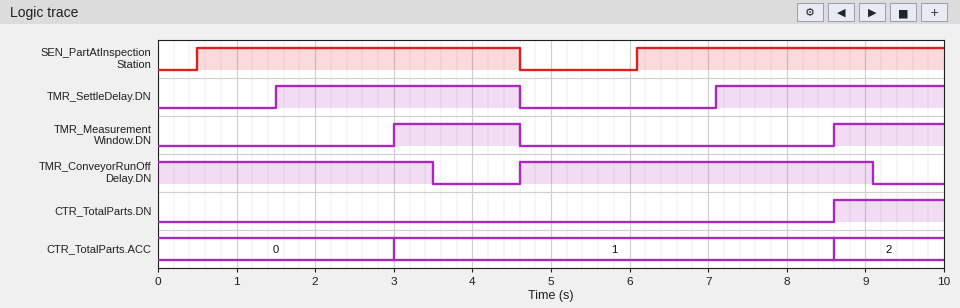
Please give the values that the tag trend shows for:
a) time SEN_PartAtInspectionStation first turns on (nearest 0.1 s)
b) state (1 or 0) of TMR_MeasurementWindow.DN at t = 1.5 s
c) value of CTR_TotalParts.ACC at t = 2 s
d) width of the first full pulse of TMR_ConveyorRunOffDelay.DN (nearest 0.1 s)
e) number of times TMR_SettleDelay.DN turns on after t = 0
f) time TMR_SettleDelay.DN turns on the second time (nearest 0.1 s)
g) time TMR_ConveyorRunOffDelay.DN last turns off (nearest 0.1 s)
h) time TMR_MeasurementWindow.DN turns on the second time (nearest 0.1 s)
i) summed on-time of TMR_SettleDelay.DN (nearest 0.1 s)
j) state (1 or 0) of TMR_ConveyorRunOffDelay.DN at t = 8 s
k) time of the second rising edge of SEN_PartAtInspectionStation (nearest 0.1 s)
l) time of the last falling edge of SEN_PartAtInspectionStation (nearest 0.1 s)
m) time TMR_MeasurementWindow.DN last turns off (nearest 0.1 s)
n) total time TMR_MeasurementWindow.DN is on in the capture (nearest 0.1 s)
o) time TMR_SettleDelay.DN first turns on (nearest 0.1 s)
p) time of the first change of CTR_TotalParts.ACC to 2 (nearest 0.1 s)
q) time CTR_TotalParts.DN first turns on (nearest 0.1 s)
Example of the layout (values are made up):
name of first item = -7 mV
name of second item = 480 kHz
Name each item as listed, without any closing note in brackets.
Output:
time SEN_PartAtInspectionStation first turns on = 0.5 s
state (1 or 0) of TMR_MeasurementWindow.DN at t = 1.5 s = 0
value of CTR_TotalParts.ACC at t = 2 s = 0
width of the first full pulse of TMR_ConveyorRunOffDelay.DN = 4.5 s
number of times TMR_SettleDelay.DN turns on after t = 0 = 2
time TMR_SettleDelay.DN turns on the second time = 7.1 s
time TMR_ConveyorRunOffDelay.DN last turns off = 9.1 s
time TMR_MeasurementWindow.DN turns on the second time = 8.6 s
summed on-time of TMR_SettleDelay.DN = 6.0 s
state (1 or 0) of TMR_ConveyorRunOffDelay.DN at t = 8 s = 1
time of the second rising edge of SEN_PartAtInspectionStation = 6.1 s
time of the last falling edge of SEN_PartAtInspectionStation = 4.6 s
time TMR_MeasurementWindow.DN last turns off = 4.6 s
total time TMR_MeasurementWindow.DN is on in the capture = 3.0 s
time TMR_SettleDelay.DN first turns on = 1.5 s
time of the first change of CTR_TotalParts.ACC to 2 = 8.6 s
time CTR_TotalParts.DN first turns on = 8.6 s
